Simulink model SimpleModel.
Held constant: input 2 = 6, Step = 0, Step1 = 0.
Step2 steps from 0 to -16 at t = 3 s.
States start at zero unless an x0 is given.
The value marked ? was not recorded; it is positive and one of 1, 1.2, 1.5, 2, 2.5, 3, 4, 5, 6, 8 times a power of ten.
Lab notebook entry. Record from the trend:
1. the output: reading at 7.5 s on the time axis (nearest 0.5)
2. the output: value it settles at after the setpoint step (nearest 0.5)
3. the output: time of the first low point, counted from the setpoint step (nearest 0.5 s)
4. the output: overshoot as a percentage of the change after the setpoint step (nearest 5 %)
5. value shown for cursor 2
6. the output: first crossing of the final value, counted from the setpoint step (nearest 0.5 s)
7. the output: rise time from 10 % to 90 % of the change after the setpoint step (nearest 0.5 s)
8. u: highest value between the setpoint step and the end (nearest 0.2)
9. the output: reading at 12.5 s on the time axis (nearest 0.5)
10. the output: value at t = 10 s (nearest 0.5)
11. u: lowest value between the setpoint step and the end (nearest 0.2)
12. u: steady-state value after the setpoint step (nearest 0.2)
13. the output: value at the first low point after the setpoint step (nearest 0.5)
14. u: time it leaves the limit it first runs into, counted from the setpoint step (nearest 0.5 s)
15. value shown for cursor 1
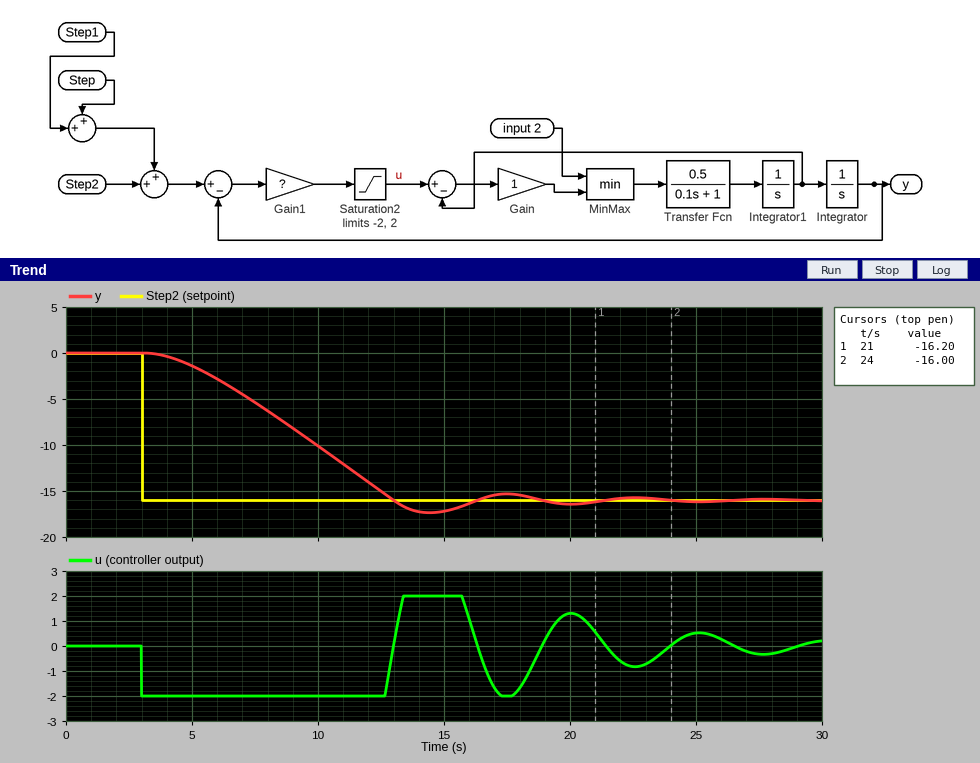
-5.5
-16.0
11.5 s
10 %
-16.00
10.0 s
7.0 s
2.0
-15.0
-10.0
-2.0
0.0
-17.5
9.5 s
-16.20
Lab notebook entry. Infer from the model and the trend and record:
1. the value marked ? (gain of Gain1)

3
